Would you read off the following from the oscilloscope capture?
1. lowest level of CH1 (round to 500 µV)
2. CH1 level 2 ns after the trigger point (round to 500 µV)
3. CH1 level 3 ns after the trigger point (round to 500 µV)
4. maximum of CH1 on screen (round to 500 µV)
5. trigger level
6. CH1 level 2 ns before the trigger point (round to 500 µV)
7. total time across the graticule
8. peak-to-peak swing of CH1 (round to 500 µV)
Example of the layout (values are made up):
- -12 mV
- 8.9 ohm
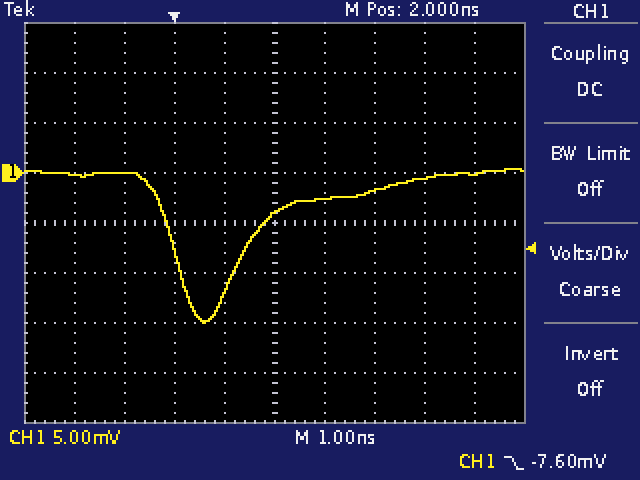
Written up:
- -15.0 mV
- -4.0 mV
- -2.5 mV
- 500 µV
- -7.60 mV
- 0.0 mV
- 10 ns
- 15.5 mV
